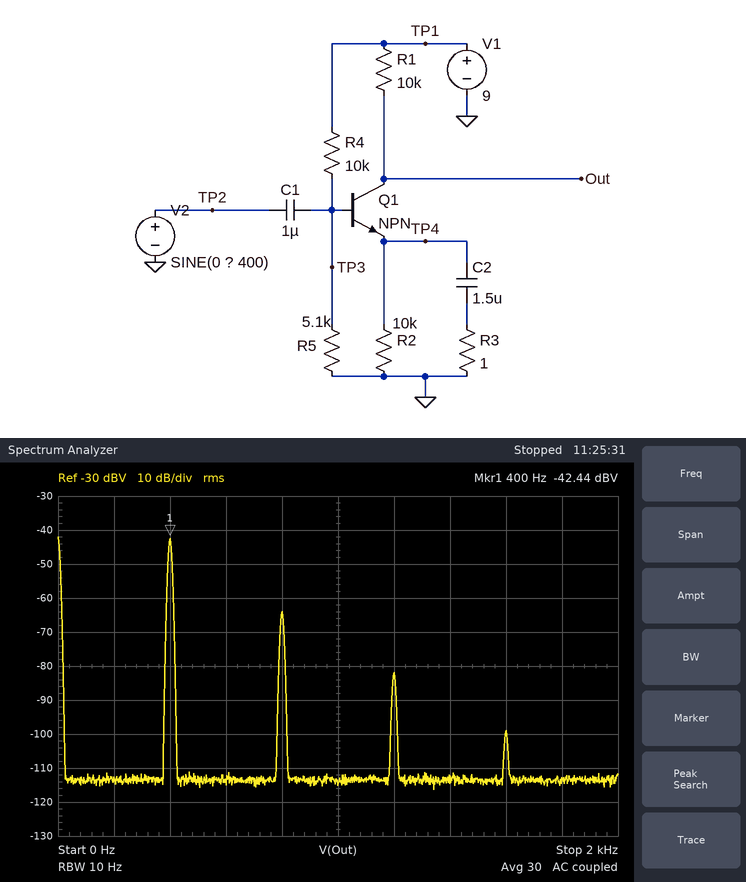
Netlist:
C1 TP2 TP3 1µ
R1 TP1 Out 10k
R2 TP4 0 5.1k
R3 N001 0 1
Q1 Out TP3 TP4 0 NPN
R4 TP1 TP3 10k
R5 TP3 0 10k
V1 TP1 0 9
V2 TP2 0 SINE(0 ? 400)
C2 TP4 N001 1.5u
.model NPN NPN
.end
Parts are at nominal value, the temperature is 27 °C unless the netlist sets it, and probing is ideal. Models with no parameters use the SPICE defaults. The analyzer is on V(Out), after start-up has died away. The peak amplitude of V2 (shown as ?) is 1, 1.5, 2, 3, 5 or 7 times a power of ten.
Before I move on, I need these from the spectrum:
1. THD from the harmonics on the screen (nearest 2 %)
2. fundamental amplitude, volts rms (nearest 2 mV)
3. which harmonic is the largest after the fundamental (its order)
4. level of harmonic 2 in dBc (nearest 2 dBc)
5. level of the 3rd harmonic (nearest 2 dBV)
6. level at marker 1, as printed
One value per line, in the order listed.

8 %
8 mV
2
-22 dBc
-82 dBV
-42.44 dBV
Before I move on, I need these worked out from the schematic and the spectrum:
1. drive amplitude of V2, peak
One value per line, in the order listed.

20 mV
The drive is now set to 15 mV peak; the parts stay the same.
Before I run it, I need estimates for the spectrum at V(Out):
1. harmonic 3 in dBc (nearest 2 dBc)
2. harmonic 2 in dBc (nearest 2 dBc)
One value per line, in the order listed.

-44 dBc
-24 dBc
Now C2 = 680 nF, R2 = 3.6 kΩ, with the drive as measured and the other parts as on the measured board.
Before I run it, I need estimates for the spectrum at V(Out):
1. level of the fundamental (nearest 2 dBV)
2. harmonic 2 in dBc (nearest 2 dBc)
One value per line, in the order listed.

-42 dBV
-42 dBc
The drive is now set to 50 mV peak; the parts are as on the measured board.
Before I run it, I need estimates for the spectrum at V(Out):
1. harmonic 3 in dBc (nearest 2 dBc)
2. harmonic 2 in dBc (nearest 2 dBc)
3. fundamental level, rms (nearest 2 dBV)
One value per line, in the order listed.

-18 dBc
-10 dBc
-32 dBV
